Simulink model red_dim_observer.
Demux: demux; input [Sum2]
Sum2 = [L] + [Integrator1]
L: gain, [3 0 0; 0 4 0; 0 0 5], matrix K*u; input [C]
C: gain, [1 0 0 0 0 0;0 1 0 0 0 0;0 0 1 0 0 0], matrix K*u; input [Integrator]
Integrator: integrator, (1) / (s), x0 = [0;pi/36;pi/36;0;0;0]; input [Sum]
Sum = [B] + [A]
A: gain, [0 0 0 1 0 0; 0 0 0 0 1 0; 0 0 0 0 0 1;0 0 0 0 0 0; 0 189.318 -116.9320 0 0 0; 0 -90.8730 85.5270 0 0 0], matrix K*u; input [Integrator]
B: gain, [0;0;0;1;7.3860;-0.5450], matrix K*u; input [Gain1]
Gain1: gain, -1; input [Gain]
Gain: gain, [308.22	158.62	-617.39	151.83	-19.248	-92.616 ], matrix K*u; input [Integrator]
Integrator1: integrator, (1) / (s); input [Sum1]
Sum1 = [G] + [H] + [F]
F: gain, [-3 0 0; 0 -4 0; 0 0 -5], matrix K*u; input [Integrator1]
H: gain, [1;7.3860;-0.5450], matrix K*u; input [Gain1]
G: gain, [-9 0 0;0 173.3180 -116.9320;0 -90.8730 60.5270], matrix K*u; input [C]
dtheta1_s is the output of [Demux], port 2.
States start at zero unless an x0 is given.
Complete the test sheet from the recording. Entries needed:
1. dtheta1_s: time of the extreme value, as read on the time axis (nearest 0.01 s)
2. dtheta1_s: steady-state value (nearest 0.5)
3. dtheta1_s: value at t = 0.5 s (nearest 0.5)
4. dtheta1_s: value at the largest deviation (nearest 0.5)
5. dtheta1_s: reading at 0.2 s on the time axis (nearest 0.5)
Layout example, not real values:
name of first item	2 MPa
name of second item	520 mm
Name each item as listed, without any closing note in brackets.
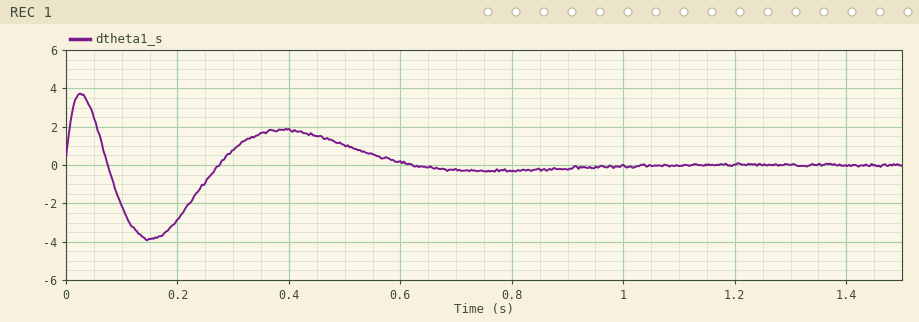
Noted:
dtheta1_s: time of the extreme value, as read on the time axis	0.15 s
dtheta1_s: steady-state value	0.0
dtheta1_s: value at t = 0.5 s	1.0
dtheta1_s: value at the largest deviation	-4.0
dtheta1_s: reading at 0.2 s on the time axis	-3.0
